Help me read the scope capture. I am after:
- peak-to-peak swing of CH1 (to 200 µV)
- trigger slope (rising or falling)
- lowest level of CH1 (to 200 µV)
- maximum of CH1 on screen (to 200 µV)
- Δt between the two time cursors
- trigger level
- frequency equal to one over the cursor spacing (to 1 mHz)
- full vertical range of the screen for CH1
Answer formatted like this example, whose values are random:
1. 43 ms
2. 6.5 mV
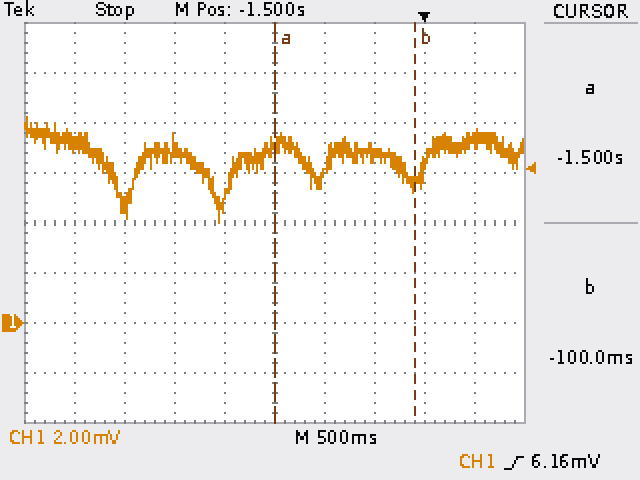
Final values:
1. 4.2 mV
2. rising
3. 4.0 mV
4. 8.2 mV
5. 1.40 s
6. 6.16 mV
7. 714 mHz
8. 16 mV
